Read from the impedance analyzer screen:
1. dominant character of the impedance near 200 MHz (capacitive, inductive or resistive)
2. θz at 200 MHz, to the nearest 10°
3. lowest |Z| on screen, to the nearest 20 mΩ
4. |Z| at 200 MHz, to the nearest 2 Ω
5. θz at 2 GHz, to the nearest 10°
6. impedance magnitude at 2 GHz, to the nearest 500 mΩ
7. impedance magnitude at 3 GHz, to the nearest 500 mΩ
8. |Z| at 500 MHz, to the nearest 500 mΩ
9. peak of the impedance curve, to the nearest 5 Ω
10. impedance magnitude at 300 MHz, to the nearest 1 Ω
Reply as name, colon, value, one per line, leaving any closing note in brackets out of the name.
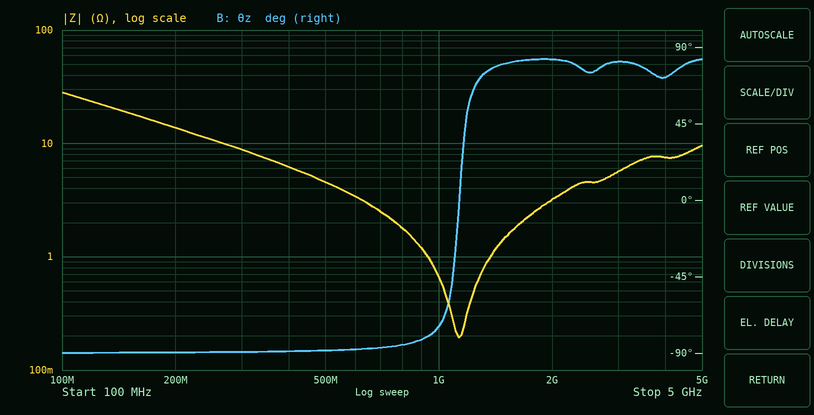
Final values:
dominant character of the impedance near 200 MHz: capacitive
θz at 200 MHz, to the nearest 10°: -90°
lowest |Z| on screen, to the nearest 20 mΩ: 200 mΩ
|Z| at 200 MHz, to the nearest 2 Ω: 14 Ω
θz at 2 GHz, to the nearest 10°: 80°
impedance magnitude at 2 GHz, to the nearest 500 mΩ: 3.0 Ω
impedance magnitude at 3 GHz, to the nearest 500 mΩ: 5.5 Ω
|Z| at 500 MHz, to the nearest 500 mΩ: 4.5 Ω
peak of the impedance curve, to the nearest 5 Ω: 30 Ω
impedance magnitude at 300 MHz, to the nearest 1 Ω: 9 Ω
